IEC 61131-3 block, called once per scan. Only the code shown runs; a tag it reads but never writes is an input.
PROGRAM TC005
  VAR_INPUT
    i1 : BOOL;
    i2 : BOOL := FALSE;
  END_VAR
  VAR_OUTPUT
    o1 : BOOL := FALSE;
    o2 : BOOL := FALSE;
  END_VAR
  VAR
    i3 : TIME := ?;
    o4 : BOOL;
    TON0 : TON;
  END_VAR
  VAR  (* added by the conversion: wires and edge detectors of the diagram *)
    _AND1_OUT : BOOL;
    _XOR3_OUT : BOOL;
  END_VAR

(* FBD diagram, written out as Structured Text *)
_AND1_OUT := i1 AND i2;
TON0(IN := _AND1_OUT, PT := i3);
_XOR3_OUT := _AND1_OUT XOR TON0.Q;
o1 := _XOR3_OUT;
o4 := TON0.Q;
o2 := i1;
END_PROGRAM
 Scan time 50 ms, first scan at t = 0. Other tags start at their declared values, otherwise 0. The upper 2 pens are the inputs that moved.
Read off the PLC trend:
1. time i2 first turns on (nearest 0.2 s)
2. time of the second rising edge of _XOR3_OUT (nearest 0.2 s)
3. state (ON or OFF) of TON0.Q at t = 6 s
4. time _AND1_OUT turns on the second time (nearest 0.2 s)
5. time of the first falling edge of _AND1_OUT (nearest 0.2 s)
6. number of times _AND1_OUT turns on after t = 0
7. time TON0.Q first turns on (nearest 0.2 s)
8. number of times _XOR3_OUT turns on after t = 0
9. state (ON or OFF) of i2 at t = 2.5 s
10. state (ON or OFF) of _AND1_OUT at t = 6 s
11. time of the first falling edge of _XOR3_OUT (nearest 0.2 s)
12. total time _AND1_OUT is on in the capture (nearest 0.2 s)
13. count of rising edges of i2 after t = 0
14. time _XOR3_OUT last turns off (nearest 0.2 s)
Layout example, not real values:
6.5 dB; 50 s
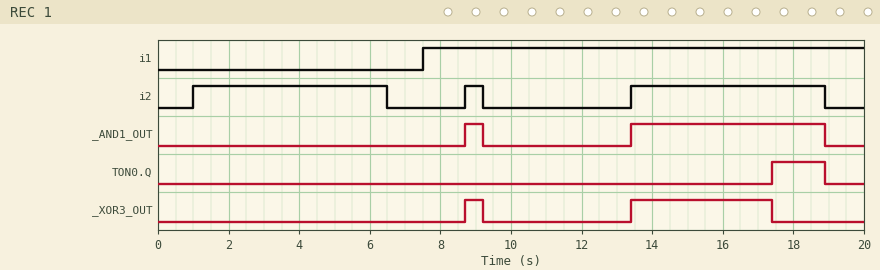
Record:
1.0 s; 13.4 s; OFF; 13.4 s; 9.2 s; 2; 17.4 s; 2; ON; OFF; 9.2 s; 6.0 s; 3; 17.4 s
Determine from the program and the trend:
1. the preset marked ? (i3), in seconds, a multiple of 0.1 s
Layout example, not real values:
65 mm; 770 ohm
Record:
4.0 s
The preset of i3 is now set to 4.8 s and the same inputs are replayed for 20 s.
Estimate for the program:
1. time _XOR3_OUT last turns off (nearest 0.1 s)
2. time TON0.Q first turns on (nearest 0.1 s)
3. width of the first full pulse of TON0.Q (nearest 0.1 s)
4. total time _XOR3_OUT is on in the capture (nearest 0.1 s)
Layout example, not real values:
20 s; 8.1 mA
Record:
18.2 s; 18.2 s; 0.7 s; 5.3 s
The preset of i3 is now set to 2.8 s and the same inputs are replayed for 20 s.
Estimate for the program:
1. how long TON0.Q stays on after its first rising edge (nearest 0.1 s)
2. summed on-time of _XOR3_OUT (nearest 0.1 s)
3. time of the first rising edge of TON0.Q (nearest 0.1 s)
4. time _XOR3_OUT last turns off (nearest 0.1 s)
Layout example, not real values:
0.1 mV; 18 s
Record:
2.7 s; 3.3 s; 16.2 s; 16.2 s
